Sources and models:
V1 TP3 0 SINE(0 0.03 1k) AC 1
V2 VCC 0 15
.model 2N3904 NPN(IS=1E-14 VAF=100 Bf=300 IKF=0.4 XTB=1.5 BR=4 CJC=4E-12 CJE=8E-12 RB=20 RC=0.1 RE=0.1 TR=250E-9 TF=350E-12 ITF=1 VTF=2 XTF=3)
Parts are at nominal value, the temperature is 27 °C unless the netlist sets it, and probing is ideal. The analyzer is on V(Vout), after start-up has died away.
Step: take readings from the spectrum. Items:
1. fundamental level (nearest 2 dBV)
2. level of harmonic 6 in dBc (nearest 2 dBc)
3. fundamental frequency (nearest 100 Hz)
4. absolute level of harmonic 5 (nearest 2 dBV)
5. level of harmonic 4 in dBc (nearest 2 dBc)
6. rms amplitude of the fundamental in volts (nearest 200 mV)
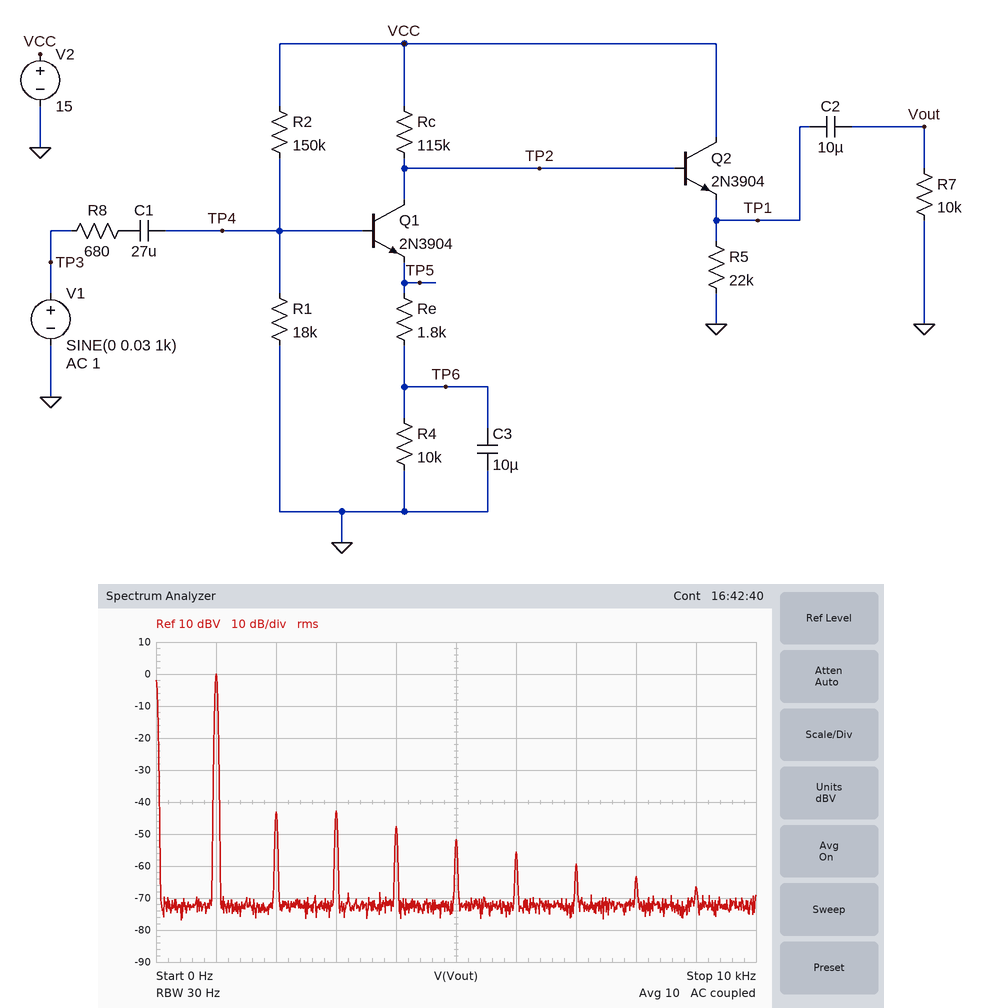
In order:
0 dBV
-56 dBc
1.0 kHz
-52 dBV
-48 dBc
1.0 V
